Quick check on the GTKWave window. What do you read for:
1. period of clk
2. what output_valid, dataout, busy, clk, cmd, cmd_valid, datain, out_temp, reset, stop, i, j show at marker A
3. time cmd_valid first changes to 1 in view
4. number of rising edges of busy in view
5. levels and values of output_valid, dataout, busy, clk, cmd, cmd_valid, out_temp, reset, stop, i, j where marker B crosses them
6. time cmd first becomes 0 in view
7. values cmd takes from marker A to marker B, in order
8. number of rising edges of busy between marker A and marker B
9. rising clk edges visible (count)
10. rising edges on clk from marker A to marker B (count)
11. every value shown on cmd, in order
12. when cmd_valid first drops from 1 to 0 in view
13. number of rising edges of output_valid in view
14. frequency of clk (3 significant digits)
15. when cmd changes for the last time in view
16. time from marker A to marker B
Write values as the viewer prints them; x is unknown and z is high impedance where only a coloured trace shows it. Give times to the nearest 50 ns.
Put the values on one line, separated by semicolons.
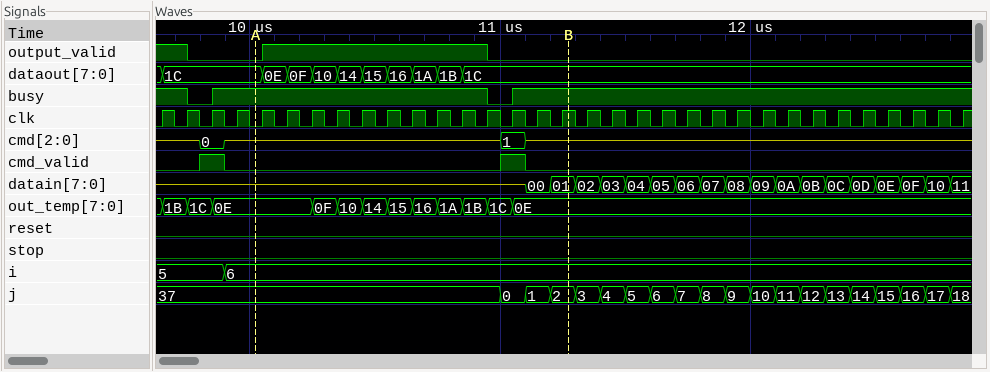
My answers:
100 ns; output_valid=0, dataout=1C, busy=1, clk=0, cmd=z, cmd_valid=0, datain=z, out_temp=0E, reset=0, stop=0, i=6, j=37; 9800 ns; 2; output_valid=0, dataout=1C, busy=1, clk=1, cmd=z, cmd_valid=0, out_temp=0E, reset=0, stop=0, i=6, j=2; 9800 ns; z, 1, z; 1; 33; 13; z, 0, z, 1, z; 9900 ns; 1; 10.0 MHz; 11100 ns; 1250 ns
